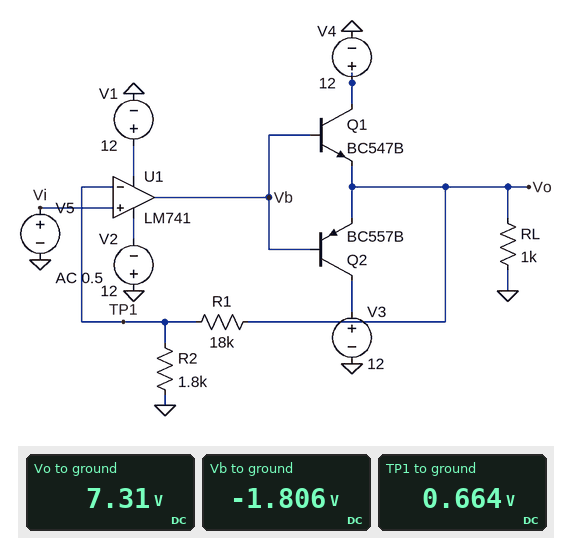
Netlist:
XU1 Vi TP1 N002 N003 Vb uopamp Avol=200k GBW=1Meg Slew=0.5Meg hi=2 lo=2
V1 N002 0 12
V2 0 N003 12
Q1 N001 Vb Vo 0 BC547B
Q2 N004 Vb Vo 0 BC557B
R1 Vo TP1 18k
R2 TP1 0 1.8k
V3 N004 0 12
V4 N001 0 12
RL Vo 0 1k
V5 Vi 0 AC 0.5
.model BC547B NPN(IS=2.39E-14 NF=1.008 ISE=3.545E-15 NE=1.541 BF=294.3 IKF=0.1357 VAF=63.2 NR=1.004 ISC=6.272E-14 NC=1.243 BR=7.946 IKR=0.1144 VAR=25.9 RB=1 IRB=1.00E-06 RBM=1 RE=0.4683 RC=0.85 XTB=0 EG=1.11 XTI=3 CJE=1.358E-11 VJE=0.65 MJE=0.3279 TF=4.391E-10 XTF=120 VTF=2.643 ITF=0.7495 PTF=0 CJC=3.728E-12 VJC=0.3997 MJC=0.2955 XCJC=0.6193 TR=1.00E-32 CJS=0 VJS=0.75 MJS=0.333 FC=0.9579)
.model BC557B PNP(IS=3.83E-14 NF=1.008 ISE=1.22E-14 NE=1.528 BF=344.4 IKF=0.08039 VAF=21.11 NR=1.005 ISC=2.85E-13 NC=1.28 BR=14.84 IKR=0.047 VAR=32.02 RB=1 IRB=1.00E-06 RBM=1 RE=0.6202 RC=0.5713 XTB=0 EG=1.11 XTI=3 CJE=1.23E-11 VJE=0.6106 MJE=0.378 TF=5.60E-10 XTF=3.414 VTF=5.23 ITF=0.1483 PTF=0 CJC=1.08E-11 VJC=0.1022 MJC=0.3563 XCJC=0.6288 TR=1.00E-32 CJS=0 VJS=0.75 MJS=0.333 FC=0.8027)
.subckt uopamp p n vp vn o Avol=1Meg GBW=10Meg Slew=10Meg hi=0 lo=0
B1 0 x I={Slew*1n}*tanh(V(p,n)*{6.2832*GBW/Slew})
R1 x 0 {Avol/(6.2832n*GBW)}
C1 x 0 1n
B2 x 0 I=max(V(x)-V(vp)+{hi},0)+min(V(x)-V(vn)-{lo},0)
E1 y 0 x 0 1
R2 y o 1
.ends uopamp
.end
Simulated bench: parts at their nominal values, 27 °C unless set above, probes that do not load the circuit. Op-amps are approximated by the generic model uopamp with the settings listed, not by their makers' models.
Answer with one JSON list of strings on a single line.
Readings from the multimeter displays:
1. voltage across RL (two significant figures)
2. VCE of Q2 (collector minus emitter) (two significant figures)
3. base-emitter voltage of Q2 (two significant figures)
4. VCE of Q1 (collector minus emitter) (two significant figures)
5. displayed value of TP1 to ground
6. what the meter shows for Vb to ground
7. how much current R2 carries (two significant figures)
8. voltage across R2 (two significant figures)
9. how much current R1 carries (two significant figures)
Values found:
["7.3 V", "4.7 V", "-9.1 V", "4.7 V", "0.664 V", "-1.806 V", "370 µA", "660 mV", "370 µA"]
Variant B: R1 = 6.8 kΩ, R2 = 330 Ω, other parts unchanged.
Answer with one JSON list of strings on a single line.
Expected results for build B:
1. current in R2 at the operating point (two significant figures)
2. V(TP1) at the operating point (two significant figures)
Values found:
["1.0 mA", "340 mV"]
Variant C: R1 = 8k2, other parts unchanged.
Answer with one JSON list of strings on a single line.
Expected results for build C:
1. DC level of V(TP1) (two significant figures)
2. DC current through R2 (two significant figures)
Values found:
["1.3 V", "730 µA"]
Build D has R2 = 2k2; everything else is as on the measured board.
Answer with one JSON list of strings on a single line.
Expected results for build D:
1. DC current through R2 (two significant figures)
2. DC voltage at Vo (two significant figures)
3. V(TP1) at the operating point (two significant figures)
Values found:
["360 µA", "7.3 V", "800 mV"]
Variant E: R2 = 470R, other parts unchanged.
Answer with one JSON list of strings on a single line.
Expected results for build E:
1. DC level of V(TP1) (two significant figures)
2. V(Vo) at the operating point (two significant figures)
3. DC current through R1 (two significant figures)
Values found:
["190 mV", "7.3 V", "400 µA"]
